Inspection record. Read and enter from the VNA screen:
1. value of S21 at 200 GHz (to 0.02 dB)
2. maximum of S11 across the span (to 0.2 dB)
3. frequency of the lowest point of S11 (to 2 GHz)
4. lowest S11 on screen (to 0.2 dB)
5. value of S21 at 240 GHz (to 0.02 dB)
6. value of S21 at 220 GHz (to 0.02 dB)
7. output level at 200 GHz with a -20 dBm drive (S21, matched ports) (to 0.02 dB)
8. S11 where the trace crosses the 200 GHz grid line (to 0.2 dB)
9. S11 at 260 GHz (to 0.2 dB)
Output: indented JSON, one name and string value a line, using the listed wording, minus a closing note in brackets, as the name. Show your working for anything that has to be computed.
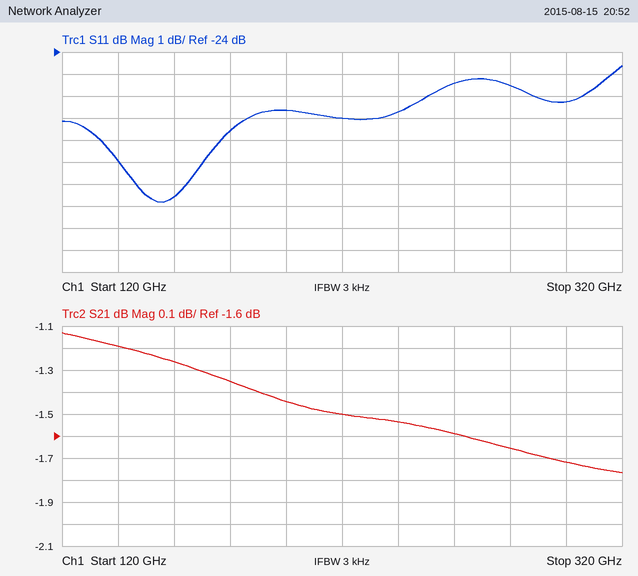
{
  "value of S21 at 200 GHz": "-1.44 dB",
  "maximum of S11 across the span": "-24.6 dB",
  "frequency of the lowest point of S11": "156 GHz",
  "lowest S11 on screen": "-30.8 dB",
  "value of S21 at 240 GHz": "-1.54 dB",
  "value of S21 at 220 GHz": "-1.50 dB",
  "output level at 200 GHz with a -20 dBm drive (S21, matched ports)": "-20 dBm + (-1.44 dB) = -21.44 dBm",
  "S11 where the trace crosses the 200 GHz grid line": "-26.6 dB",
  "S11 at 260 GHz": "-25.4 dB"
}
